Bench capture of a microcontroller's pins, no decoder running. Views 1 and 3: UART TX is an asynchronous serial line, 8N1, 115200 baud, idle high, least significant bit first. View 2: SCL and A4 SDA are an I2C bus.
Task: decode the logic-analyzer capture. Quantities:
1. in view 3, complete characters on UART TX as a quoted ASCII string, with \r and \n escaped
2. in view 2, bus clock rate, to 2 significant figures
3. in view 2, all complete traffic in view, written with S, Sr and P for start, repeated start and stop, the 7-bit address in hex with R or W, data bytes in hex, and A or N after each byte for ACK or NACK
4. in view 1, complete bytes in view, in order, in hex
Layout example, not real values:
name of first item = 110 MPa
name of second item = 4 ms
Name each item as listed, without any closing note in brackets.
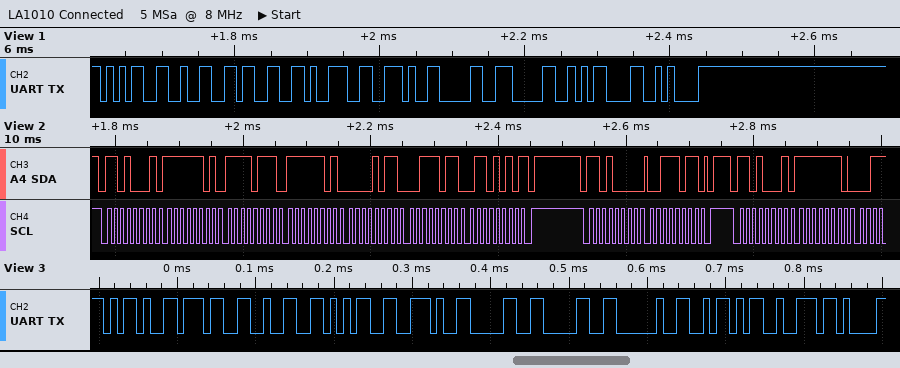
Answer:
in view 3, complete characters on UART TX as a quoted ASCII string, with \r and \n escaped = "-725.00 Zr"
in view 2, bus clock rate, to 2 significant figures = 100 kHz
in view 2, all complete traffic in view, written with S, Sr and P for start, repeated start and stop, the 7-bit address in hex with R or W, data bytes in hex, and A or N after each byte for ACK or NACK = S 68R A FD A F7 A FD A 0B A 3B A 6A N P S 68W A 3B A P S 68R A FE A
in view 1, complete bytes in view, in order, in hex = 0x35 0x32 0x33 0x39 0x2E 0x30 0x30 0x0D 0x0A
